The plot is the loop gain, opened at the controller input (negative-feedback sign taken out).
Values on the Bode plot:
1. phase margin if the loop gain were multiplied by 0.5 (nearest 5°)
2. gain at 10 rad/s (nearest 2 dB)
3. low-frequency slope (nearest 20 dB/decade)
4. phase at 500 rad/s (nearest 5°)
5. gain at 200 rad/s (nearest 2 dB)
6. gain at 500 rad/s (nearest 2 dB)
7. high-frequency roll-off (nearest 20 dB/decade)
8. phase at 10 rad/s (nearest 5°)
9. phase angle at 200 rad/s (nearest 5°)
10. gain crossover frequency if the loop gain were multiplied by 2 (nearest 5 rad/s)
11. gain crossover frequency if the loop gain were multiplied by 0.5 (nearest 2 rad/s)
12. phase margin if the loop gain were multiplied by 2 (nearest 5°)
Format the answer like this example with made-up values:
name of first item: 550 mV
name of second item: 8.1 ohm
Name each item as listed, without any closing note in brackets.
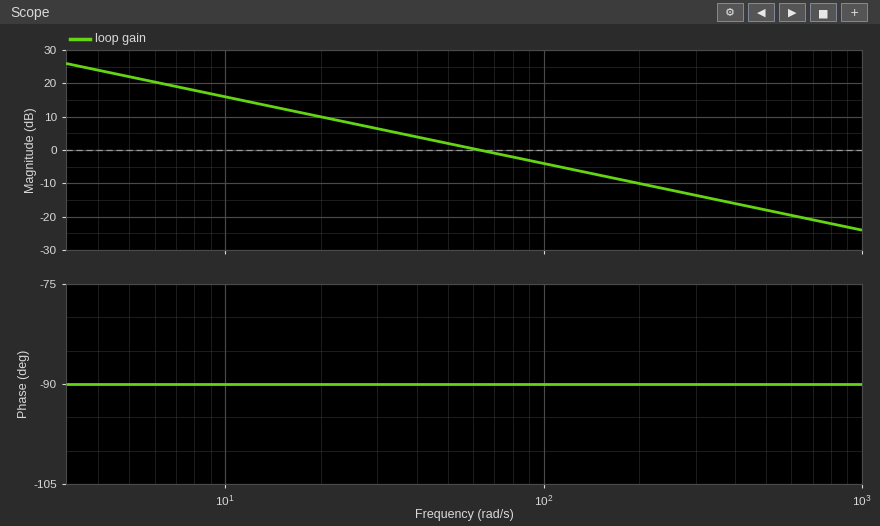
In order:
phase margin if the loop gain were multiplied by 0.5: 90°
gain at 10 rad/s: 16 dB
low-frequency slope: -20 dB/decade
phase at 500 rad/s: -90°
gain at 200 rad/s: -10 dB
gain at 500 rad/s: -18 dB
high-frequency roll-off: -20 dB/decade
phase at 10 rad/s: -90°
phase angle at 200 rad/s: -90°
gain crossover frequency if the loop gain were multiplied by 2: 125 rad/s
gain crossover frequency if the loop gain were multiplied by 0.5: 32 rad/s
phase margin if the loop gain were multiplied by 2: 90°
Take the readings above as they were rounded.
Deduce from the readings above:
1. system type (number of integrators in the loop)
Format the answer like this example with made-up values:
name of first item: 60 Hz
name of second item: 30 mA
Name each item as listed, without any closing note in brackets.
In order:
system type: 1
